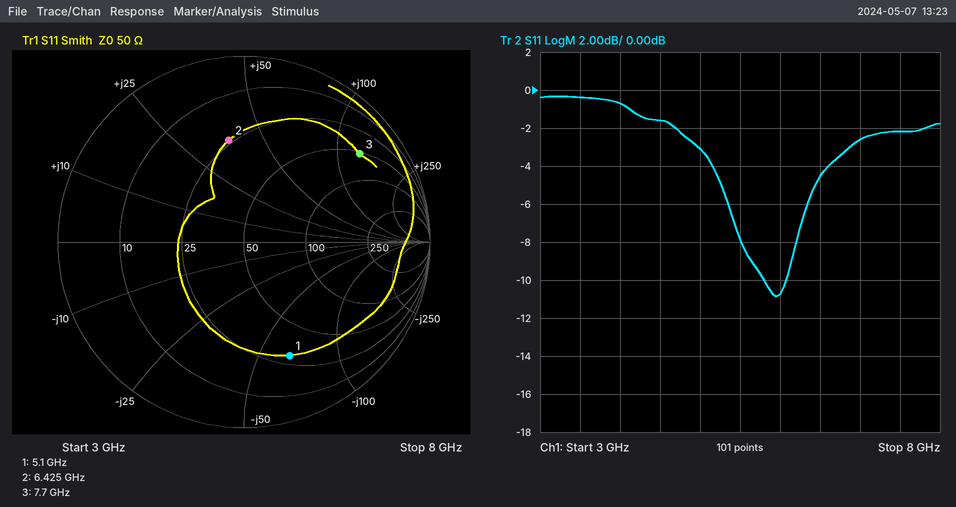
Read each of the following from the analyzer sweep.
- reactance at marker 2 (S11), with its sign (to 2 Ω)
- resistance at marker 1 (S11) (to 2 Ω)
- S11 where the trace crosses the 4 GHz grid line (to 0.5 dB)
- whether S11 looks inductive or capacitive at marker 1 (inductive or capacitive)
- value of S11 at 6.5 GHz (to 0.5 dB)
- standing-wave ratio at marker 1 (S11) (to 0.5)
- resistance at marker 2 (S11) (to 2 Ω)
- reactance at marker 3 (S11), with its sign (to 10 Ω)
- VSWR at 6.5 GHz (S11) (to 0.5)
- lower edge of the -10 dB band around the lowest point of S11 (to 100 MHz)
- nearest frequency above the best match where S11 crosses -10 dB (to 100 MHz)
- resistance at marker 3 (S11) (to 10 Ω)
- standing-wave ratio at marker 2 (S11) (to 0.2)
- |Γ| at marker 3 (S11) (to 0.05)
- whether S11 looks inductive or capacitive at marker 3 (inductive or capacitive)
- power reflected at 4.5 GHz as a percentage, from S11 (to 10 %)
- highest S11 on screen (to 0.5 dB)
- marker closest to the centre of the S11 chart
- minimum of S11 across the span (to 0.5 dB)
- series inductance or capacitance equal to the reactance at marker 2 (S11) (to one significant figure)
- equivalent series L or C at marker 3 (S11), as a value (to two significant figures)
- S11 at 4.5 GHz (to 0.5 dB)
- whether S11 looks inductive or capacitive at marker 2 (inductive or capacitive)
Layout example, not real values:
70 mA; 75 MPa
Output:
+38 Ω; 30 Ω; -0.5 dB; capacitive; -4.5 dB; 5.0; 24 Ω; +130 Ω; 4.0; 5.8 GHz; 6.1 GHz; 50 Ω; 3.4; 0.80; inductive; 70 %; -0.5 dB; marker 2; -11.0 dB; 900 pH; 2.7 nH; -1.5 dB; inductive
